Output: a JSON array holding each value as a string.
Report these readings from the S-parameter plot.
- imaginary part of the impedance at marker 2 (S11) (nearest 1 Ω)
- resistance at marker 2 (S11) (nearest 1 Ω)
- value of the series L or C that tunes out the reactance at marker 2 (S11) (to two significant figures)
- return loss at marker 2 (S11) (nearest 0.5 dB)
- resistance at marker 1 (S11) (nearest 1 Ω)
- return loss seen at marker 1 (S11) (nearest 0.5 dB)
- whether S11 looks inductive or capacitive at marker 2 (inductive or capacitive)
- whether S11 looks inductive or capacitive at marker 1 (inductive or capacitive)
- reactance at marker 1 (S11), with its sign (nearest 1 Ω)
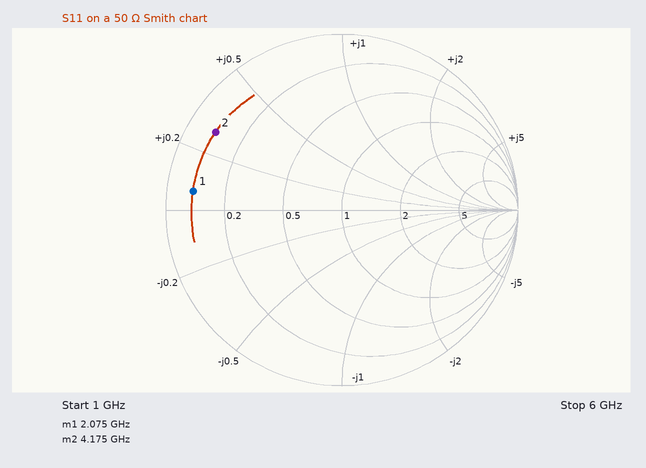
["+14 Ω", "5 Ω", "2.7 pF", "1.5 dB", "4 Ω", "1.5 dB", "inductive", "inductive", "+3 Ω"]
